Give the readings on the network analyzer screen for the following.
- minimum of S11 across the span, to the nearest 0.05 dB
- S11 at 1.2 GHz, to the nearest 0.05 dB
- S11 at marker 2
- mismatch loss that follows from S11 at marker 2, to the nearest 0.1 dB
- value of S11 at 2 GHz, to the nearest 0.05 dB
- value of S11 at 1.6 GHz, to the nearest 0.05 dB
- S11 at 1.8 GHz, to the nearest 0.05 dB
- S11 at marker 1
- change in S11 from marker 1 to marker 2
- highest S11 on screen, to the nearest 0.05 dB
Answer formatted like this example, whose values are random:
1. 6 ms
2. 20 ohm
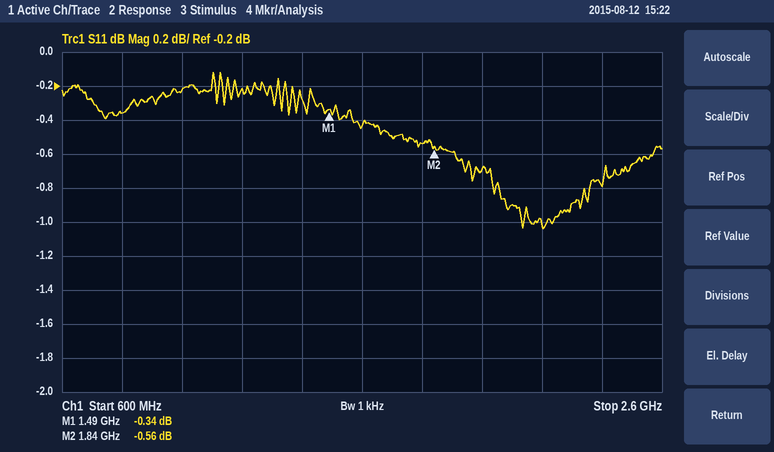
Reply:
1. -1.05 dB
2. -0.20 dB
3. -0.56 dB
4. 9.2 dB
5. -0.70 dB
6. -0.45 dB
7. -0.55 dB
8. -0.34 dB
9. -0.22 dB
10. -0.10 dB
